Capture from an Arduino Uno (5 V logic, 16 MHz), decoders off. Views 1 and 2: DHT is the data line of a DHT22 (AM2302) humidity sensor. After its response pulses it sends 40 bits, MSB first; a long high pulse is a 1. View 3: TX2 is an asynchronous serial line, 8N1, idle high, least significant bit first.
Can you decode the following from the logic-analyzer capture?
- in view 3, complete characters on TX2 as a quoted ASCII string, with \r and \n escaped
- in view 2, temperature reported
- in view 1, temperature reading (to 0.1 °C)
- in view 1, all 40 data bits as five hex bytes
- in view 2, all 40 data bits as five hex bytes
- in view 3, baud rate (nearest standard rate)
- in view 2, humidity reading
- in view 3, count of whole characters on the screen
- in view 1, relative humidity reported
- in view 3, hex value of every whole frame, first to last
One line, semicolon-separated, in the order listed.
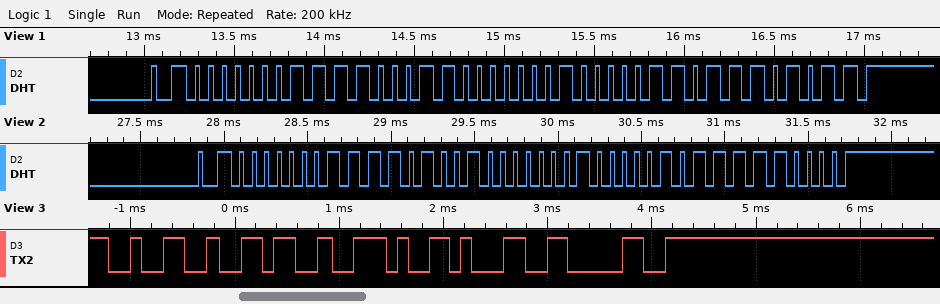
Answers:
"26.10"; 26.1 °C; 26.2 °C; 01 E3 01 06 EB; 01 E9 01 05 F0; 9600 baud; 48.9 %; 5; 48.3 %; 32 36 2E 31 30
